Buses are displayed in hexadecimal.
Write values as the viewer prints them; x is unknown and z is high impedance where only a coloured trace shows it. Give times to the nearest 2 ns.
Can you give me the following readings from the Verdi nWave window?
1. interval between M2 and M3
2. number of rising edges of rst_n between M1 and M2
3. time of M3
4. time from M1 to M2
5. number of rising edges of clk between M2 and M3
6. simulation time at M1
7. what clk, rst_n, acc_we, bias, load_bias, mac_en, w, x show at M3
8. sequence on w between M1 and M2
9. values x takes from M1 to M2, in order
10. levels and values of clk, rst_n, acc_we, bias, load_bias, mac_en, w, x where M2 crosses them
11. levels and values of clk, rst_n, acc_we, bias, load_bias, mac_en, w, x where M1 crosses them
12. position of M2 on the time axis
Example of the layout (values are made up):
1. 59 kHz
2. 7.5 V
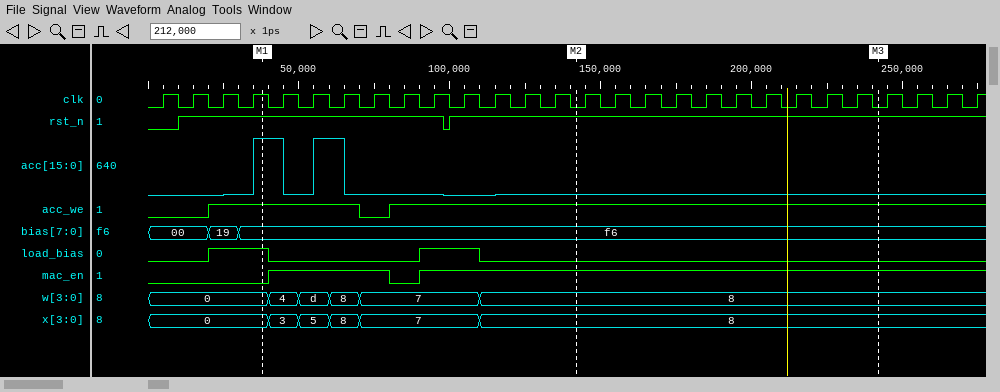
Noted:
1. 100 ns
2. 1
3. 242 ns
4. 104 ns
5. 10
6. 38 ns
7. clk=0, rst_n=1, acc_we=1, bias=f6, load_bias=0, mac_en=1, w=8, x=8
8. 0, 4, d, 8, 7, 8
9. 0, 3, 5, 8, 7, 8
10. clk=0, rst_n=1, acc_we=1, bias=f6, load_bias=0, mac_en=1, w=8, x=8
11. clk=1, rst_n=1, acc_we=1, bias=f6, load_bias=1, mac_en=0, w=0, x=0
12. 142 ns
